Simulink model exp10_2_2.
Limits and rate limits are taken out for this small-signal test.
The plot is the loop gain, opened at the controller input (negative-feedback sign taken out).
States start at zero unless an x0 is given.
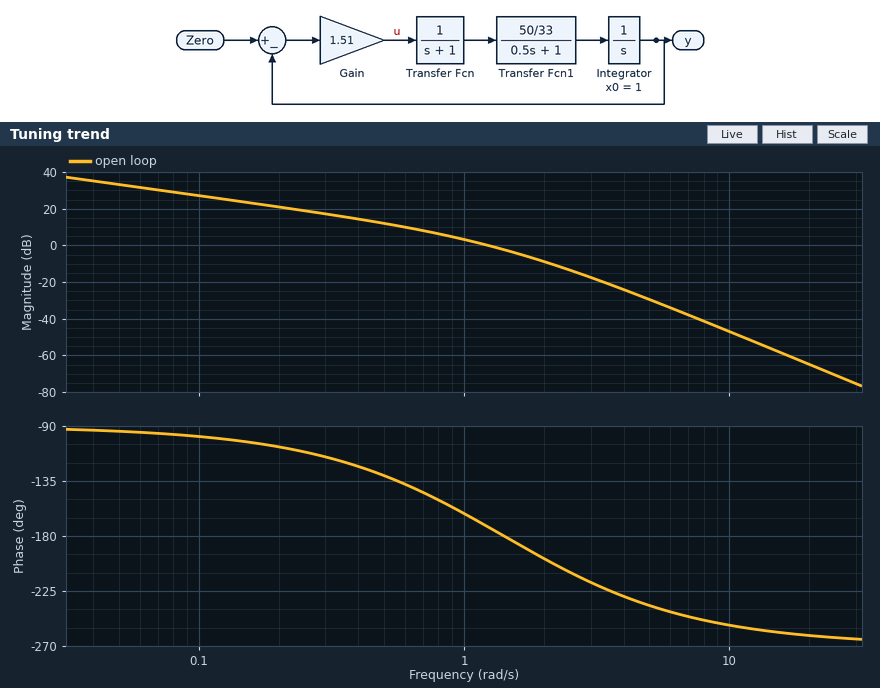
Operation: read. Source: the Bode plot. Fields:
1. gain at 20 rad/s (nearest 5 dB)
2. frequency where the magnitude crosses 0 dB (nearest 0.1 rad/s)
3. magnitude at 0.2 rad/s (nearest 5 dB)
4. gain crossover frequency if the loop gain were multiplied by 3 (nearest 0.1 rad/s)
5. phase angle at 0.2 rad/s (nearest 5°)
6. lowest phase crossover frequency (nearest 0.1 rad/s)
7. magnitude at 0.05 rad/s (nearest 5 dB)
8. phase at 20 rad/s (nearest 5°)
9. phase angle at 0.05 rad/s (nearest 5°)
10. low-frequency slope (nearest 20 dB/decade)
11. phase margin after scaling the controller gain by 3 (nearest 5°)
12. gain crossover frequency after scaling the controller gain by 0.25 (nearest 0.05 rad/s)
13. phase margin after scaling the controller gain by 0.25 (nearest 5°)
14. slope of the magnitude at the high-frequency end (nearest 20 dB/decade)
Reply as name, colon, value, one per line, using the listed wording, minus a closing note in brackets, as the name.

gain at 20 rad/s: -65 dB
frequency where the magnitude crosses 0 dB: 1.2 rad/s
magnitude at 0.2 rad/s: 20 dB
gain crossover frequency if the loop gain were multiplied by 3: 2.1 rad/s
phase angle at 0.2 rad/s: -105°
lowest phase crossover frequency: 1.4 rad/s
magnitude at 0.05 rad/s: 35 dB
phase at 20 rad/s: -260°
phase angle at 0.05 rad/s: -95°
low-frequency slope: -20 dB/decade
phase margin after scaling the controller gain by 3: -20°
gain crossover frequency after scaling the controller gain by 0.25: 0.50 rad/s
phase margin after scaling the controller gain by 0.25: 50°
slope of the magnitude at the high-frequency end: -60 dB/decade
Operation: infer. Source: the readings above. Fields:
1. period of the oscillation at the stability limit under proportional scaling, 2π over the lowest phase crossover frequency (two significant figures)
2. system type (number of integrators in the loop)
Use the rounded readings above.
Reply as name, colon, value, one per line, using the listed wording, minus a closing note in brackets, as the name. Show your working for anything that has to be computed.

period of the oscillation at the stability limit under proportional scaling, 2π over the lowest phase crossover frequency: 2π / 1.4 = 4.5 s
system type: 1
